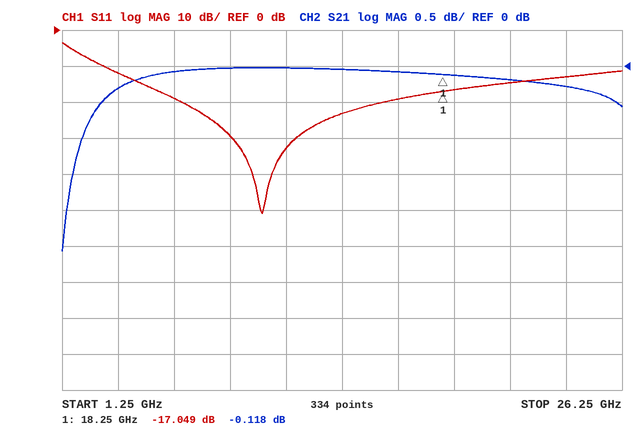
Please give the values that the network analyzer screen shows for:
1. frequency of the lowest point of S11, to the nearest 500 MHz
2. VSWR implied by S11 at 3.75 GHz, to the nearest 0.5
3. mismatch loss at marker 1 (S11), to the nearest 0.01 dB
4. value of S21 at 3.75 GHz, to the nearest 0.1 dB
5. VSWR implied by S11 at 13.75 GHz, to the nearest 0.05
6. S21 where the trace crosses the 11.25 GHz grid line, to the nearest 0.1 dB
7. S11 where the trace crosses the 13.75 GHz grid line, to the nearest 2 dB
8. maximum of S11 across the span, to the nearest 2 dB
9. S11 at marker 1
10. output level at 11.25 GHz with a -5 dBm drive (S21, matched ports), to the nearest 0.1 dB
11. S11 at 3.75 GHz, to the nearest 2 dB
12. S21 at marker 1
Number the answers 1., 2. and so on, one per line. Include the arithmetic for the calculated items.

1. 10.0 GHz
2. |Γ| = 10^(-12/20) = 0.2512; VSWR = (1 + 0.2512)/(1 − 0.2512) ≈ 1.67, so 1.5 to the nearest 0.5
3. −10 log10(1 − 10^(-17.049/10)) ≈ 0.09 dB
4. -0.3 dB
5. |Γ| = 10^(-24/20) = 0.0631; VSWR = (1 + 0.0631)/(1 − 0.0631) ≈ 1.13, so 1.15 to the nearest 0.05
6. 0.0 dB
7. -24 dB
8. -4 dB
9. -17.049 dB
10. -5 dBm + (0.0 dB) = -5.0 dBm
11. -12 dB
12. -0.118 dB
